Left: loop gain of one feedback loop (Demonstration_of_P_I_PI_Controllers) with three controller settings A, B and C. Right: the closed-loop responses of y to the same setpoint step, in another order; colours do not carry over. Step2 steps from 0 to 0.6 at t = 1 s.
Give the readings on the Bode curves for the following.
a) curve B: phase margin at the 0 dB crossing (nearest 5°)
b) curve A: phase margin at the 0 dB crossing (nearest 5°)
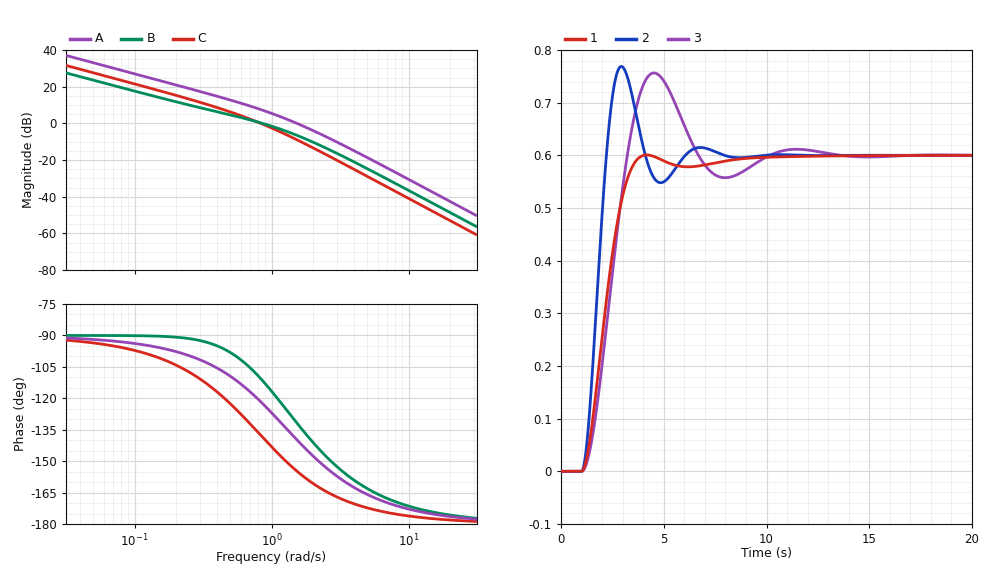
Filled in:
70°
40°
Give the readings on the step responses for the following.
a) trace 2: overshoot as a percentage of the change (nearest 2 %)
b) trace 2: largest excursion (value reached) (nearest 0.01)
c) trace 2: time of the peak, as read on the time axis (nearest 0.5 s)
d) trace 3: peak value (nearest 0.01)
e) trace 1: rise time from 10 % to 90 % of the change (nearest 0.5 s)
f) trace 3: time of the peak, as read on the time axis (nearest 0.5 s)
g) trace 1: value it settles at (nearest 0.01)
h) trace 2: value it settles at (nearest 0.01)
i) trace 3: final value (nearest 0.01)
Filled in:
28 %
0.77
3.0 s
0.76
1.5 s
4.5 s
0.60
0.60
0.60
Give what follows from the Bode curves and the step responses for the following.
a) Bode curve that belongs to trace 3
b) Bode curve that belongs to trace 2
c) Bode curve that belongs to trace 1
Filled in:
C
A
B
